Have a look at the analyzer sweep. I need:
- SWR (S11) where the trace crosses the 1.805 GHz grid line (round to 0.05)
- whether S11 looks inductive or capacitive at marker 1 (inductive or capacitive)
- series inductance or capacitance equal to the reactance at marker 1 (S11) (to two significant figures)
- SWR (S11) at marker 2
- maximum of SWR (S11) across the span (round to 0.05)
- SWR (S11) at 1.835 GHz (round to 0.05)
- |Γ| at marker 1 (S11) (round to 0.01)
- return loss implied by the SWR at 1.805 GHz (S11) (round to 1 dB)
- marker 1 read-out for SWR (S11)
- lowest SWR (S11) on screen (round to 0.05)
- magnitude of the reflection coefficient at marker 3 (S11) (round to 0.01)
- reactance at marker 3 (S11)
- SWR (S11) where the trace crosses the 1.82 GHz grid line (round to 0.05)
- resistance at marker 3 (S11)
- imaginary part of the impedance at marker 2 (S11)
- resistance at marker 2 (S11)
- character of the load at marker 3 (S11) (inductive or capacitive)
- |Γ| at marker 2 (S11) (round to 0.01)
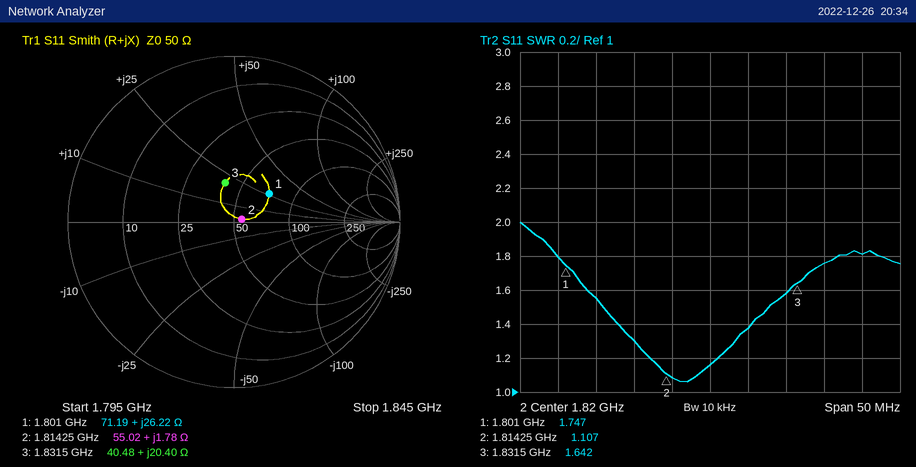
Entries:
1.55
inductive
2.3 nH
1.107
2.00
1.75
0.27
13 dB
1.747
1.05
0.24
+20.40 Ω
1.15
40.48 Ω
+1.78 Ω
55.02 Ω
inductive
0.05
